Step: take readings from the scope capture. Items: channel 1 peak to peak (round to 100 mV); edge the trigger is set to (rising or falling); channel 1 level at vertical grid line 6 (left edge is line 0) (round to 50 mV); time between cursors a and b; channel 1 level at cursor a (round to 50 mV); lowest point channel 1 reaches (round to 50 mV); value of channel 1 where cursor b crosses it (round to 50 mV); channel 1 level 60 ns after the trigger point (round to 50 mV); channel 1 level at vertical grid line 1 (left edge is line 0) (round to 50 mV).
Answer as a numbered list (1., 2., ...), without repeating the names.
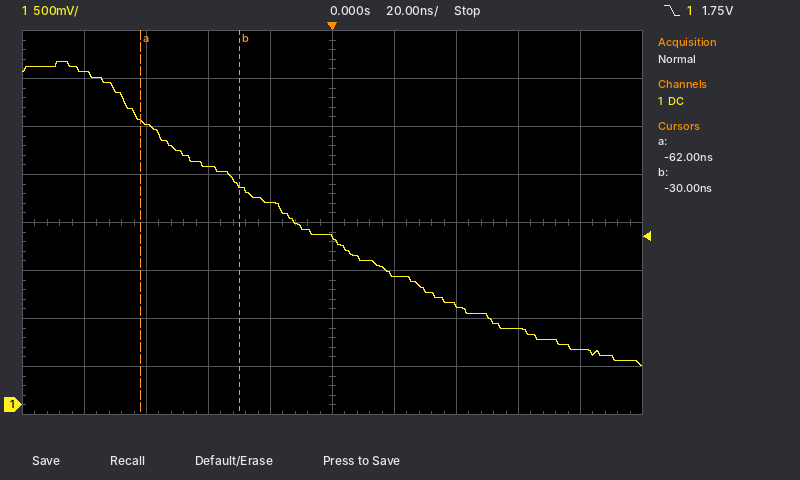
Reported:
1. 3.20 V
2. falling
3. 1.35 V
4. 32 ns
5. 2.95 V
6. 400 mV
7. 2.30 V
8. 800 mV
9. 3.45 V
